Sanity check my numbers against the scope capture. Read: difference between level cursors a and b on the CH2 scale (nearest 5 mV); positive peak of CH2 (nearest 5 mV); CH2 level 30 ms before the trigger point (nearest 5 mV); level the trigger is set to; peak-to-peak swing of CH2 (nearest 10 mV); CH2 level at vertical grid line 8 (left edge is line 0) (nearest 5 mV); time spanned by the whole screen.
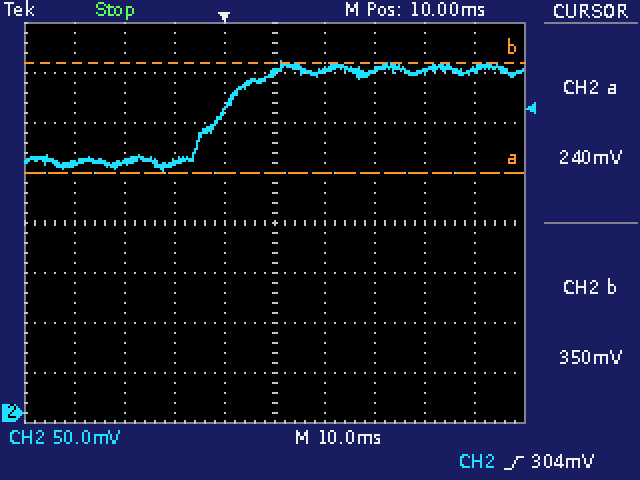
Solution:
110 mV
350 mV
250 mV
304 mV
110 mV
340 mV
100 ms
